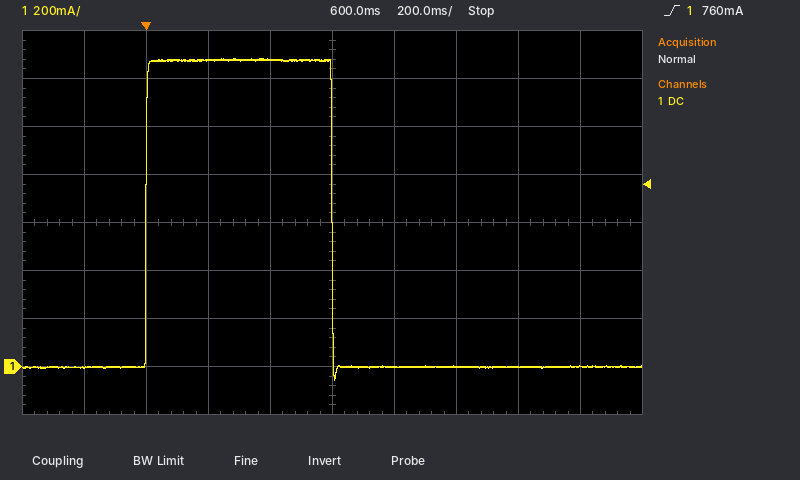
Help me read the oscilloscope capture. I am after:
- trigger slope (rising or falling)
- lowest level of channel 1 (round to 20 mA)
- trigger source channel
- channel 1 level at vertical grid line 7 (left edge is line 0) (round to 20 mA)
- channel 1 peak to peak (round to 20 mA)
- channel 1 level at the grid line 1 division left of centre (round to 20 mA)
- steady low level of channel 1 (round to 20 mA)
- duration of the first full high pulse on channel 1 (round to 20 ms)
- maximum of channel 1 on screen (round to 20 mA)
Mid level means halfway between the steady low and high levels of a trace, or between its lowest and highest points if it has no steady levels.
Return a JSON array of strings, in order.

["rising", "-60 mA", "channel 1", "0 mA", "1.34 A", "1.28 A", "0 mA", "600 ms", "1.28 A"]
